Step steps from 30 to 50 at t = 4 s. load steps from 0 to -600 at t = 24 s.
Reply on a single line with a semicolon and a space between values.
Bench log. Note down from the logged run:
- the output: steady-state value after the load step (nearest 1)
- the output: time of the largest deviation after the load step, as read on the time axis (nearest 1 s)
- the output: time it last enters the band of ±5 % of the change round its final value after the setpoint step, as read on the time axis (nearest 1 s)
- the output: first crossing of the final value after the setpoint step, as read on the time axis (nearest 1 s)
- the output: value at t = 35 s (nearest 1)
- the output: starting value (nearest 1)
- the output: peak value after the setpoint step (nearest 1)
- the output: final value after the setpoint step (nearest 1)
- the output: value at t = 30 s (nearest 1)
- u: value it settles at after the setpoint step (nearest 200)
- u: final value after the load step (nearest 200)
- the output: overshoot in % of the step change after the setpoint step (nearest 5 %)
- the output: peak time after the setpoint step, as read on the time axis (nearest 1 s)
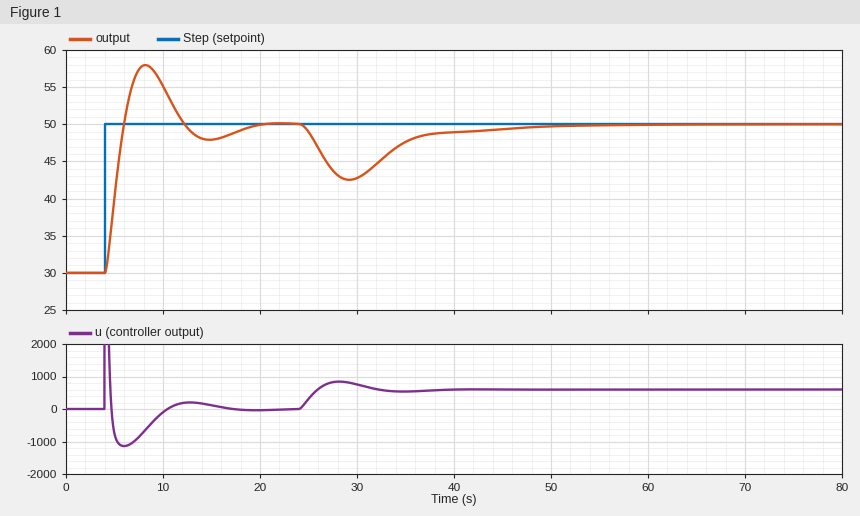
50; 29 s; 18 s; 6 s; 48; 30; 58; 50; 43; 0; 600; 40 %; 8 s
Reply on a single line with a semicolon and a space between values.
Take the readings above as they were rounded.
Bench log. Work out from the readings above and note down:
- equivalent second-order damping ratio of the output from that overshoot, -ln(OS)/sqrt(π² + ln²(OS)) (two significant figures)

0.28
